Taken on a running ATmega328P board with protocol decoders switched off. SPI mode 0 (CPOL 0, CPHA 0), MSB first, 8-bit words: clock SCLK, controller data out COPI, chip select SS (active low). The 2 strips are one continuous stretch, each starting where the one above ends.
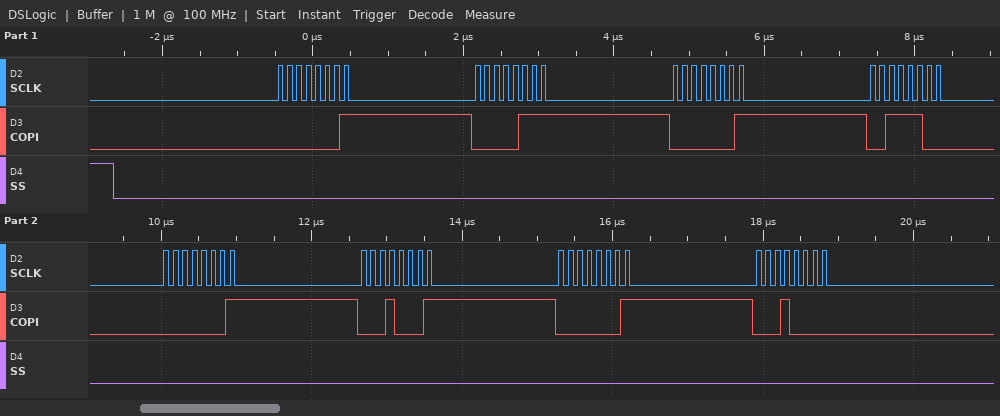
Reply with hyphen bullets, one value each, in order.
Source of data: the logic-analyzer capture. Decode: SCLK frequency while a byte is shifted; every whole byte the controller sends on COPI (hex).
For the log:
- 8 MHz
- 01 07 01 3C 01 11 01 10
